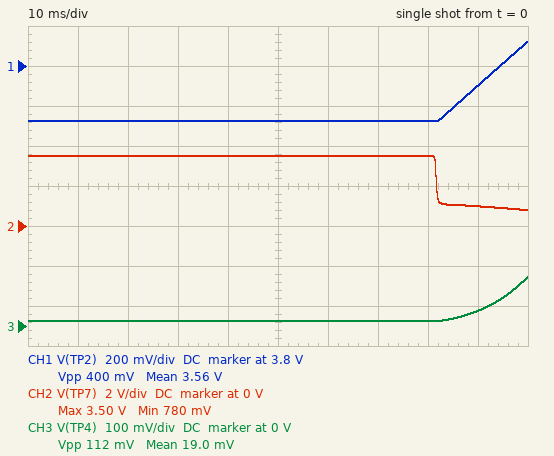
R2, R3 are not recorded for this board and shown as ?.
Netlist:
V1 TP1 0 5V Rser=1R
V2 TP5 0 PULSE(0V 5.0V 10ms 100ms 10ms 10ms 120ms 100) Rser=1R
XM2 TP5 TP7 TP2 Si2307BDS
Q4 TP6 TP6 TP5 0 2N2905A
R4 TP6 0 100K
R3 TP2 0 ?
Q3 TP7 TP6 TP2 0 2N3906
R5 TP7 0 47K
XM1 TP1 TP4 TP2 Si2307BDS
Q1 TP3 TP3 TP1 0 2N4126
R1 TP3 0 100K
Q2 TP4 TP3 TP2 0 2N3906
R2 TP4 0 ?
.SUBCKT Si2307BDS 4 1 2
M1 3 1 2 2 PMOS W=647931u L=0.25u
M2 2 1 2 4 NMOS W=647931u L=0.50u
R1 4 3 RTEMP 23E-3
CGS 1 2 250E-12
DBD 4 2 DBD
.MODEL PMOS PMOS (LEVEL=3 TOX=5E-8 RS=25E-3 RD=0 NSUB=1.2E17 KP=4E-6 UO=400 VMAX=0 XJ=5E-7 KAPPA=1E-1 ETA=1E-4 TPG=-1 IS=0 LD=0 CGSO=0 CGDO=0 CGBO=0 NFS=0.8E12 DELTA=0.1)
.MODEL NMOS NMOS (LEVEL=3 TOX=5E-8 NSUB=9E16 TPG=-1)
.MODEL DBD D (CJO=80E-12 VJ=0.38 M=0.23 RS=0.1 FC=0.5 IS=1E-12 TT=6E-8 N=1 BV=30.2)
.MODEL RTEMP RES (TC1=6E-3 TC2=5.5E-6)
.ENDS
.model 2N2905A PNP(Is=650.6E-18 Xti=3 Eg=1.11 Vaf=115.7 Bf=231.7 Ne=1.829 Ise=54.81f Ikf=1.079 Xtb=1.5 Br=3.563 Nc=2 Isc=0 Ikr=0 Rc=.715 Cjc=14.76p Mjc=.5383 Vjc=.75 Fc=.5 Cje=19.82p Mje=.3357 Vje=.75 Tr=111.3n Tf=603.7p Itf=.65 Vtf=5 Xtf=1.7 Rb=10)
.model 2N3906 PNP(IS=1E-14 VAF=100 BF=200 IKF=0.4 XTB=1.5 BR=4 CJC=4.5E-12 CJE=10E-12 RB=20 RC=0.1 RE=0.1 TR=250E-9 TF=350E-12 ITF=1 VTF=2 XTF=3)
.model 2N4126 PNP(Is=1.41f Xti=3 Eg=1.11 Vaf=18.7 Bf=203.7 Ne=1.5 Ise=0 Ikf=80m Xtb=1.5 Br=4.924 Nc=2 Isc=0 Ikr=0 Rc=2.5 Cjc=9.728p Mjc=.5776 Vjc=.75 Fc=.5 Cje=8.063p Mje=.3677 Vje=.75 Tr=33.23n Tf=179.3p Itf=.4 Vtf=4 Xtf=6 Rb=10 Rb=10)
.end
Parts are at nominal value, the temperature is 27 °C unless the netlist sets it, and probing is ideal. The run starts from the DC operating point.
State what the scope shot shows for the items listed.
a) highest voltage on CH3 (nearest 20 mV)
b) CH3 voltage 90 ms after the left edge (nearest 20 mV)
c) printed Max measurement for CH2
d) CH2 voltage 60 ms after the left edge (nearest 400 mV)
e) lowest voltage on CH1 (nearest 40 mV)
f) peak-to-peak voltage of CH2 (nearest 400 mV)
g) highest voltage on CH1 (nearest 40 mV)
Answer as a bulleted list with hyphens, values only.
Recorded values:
- 120 mV
- 40 mV
- 3.50 V
- 3.6 V
- 3.52 V
- 2.8 V
- 3.92 V
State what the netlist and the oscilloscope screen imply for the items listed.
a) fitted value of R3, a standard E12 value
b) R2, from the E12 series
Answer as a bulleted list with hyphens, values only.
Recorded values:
- 2.7 Ω
- 39 kΩ
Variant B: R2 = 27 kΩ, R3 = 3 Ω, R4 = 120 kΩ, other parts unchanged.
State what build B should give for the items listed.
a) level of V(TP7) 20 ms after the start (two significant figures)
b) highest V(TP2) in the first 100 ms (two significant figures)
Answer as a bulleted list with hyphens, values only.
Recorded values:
- 3.6 V
- 4.0 V
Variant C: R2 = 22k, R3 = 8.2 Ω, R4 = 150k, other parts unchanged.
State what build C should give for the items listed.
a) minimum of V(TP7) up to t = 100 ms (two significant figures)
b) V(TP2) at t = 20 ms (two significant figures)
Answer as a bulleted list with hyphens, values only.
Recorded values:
- 2.0 V
- 4.4 V
